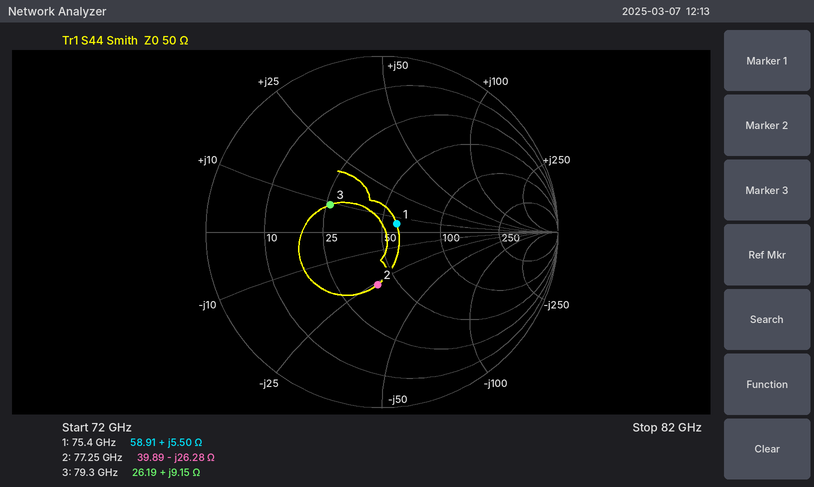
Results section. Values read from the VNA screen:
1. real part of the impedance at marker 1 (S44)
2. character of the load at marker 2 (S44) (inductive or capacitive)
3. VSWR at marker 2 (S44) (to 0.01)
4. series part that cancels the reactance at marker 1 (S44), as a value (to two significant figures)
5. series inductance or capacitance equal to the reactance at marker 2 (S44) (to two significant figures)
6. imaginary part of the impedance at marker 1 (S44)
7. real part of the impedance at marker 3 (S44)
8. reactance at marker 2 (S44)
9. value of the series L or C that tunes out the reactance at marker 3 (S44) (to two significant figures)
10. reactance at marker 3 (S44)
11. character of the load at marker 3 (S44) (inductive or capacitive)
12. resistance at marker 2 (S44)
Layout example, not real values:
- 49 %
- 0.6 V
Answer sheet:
- 58.91 Ω
- capacitive
- 1.86
- 380 fF
- 78 fF
- +5.50 Ω
- 26.19 Ω
- -26.28 Ω
- 220 fF
- +9.15 Ω
- inductive
- 39.89 Ω
